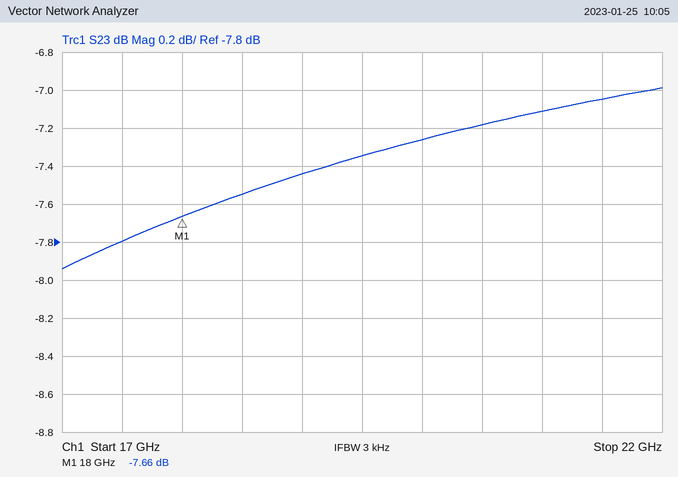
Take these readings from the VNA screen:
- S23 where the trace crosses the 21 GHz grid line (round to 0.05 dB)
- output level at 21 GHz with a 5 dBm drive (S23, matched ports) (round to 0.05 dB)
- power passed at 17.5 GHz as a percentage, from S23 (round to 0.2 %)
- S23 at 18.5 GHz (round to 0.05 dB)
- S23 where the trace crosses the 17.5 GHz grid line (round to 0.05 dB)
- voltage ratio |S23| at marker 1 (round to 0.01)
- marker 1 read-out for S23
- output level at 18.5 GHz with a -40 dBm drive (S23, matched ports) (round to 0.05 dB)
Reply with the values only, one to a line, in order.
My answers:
-7.10 dB
-2.10 dBm
16.6 %
-7.55 dB
-7.80 dB
0.41
-7.66 dB
-47.55 dBm
